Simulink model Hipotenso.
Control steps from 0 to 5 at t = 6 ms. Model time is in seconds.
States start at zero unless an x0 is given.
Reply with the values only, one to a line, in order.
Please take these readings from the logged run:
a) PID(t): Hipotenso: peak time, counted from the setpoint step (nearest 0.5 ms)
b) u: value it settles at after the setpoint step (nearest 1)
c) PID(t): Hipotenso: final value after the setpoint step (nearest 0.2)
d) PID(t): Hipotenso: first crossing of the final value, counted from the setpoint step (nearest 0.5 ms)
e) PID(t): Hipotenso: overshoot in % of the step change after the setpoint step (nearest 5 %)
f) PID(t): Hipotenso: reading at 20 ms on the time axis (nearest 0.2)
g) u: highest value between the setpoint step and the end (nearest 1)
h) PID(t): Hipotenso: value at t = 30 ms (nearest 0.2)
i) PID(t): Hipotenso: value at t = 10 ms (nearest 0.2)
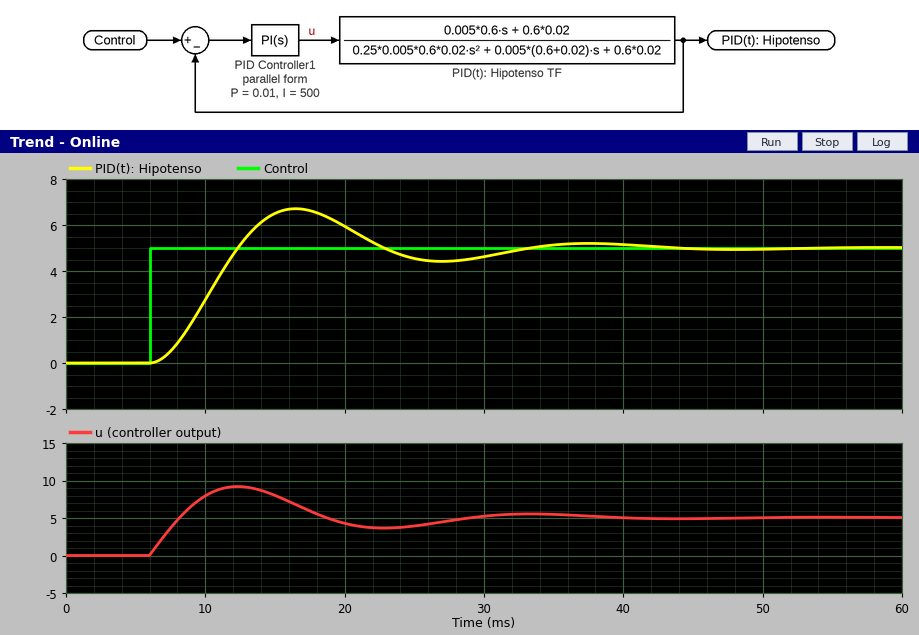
10.5 ms
5
5.0
6.5 ms
35 %
6.0
9
4.6
2.8
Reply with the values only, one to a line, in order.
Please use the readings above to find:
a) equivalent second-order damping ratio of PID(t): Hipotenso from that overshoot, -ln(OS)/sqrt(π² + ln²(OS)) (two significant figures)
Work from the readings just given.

0.32
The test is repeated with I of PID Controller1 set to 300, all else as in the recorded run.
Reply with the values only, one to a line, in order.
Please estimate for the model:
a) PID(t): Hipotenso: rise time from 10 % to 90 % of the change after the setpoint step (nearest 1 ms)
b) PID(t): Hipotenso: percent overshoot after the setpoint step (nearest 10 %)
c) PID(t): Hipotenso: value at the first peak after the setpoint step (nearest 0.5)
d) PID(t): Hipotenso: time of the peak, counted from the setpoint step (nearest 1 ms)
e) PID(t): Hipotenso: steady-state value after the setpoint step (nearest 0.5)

6 ms
20 %
6.0
14 ms
5.0
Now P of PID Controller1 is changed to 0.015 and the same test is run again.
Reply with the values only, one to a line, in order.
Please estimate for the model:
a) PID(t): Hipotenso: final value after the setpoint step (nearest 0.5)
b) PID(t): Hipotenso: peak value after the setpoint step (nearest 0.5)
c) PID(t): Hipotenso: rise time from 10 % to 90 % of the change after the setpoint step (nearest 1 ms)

5.0
6.5
4 ms
